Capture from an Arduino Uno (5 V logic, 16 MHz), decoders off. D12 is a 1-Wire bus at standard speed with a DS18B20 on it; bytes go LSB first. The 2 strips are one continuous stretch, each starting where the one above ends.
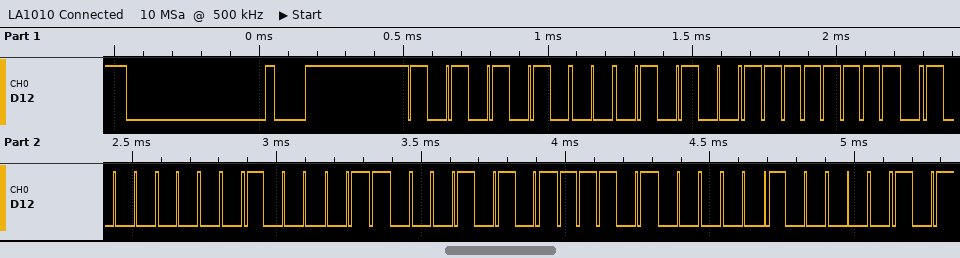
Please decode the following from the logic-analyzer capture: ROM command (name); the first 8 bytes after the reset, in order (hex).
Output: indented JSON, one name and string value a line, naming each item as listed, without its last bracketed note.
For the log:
{
  "ROM command": "Match ROM",
  "the first 8 bytes after the reset, in order": "55 28 FF 02 C2 A8 17 04"
}
